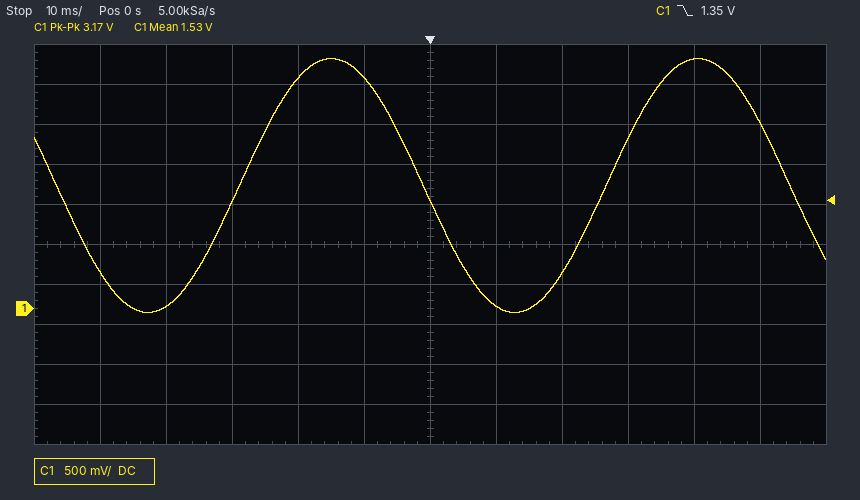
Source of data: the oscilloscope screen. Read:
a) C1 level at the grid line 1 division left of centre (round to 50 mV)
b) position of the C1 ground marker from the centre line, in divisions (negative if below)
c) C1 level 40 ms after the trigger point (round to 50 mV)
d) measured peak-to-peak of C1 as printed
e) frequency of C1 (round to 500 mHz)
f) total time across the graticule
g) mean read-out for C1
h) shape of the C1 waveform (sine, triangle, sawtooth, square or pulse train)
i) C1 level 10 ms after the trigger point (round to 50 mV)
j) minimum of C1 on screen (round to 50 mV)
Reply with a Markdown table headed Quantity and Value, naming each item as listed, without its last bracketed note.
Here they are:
| Quantity | Value |
|---|---|
| C1 level at the grid line 1 division left of centre | 2.90 V |
| position of the C1 ground marker from the centre line, in divisions | -1.6 div |
| C1 level 40 ms after the trigger point | 3.10 V |
| measured peak-to-peak of C1 as printed | 3.17 V |
| frequency of C1 | 18.0 Hz |
| total time across the graticule | 120 ms |
| mean read-out for C1 | 1.53 V |
| shape of the C1 waveform | sine |
| C1 level 10 ms after the trigger point | 50 mV |
| minimum of C1 on screen | -50 mV |
